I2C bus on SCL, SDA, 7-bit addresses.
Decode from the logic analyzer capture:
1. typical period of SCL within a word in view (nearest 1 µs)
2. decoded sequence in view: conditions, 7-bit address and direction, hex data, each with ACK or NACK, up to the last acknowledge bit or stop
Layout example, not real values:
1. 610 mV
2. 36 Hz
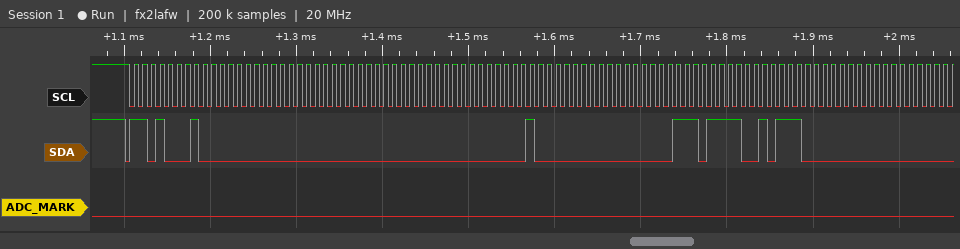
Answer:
1. 10 µs
2. start, address 68 read ACK, 00 ACK, 00 ACK, 00 ACK, 00 ACK, 40 ACK, 00 ACK, EF ACK, 5C ACK, 00 ACK
